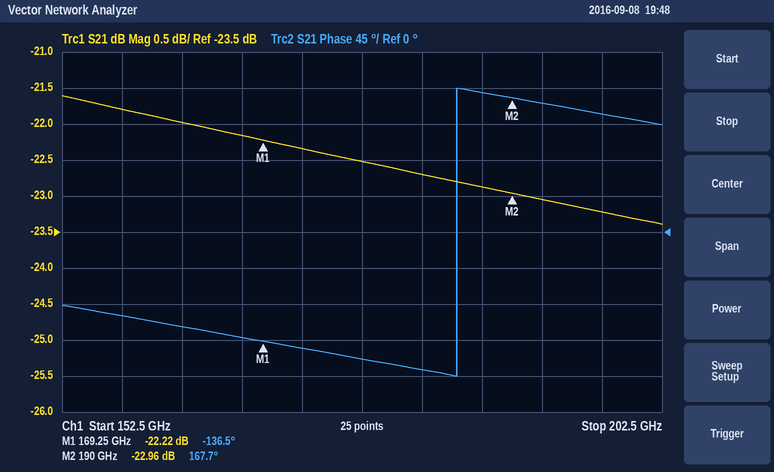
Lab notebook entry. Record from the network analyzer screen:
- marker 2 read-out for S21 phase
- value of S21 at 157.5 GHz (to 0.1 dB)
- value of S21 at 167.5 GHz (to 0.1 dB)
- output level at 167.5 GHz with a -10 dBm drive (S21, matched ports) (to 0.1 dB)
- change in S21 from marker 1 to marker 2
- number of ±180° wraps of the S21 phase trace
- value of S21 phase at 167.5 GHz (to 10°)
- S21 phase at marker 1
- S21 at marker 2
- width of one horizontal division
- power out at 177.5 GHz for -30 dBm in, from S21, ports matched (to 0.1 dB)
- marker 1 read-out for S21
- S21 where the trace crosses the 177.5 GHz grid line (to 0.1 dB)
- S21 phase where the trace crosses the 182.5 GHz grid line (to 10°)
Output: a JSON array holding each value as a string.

["167.7°", "-21.8 dB", "-22.2 dB", "-32.2 dBm", "-0.74 dB", "1", "-130°", "-136.5°", "-22.96 dB", "5 GHz", "-52.5 dBm", "-22.22 dB", "-22.5 dB", "-170°"]
